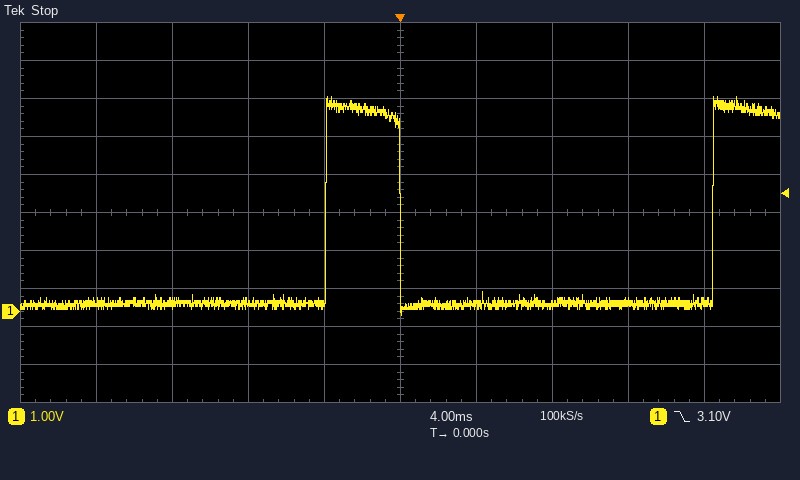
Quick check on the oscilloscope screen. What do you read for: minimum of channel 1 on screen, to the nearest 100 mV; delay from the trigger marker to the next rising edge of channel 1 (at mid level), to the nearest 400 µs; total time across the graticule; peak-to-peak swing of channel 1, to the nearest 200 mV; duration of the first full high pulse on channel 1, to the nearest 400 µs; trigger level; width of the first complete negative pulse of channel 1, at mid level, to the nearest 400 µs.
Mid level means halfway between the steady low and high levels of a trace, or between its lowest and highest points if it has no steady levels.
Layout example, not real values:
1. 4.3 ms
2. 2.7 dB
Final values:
1. -100 mV
2. 16.4 ms
3. 40 ms
4. 5.8 V
5. 4.0 ms
6. 3.10 V
7. 16.4 ms
